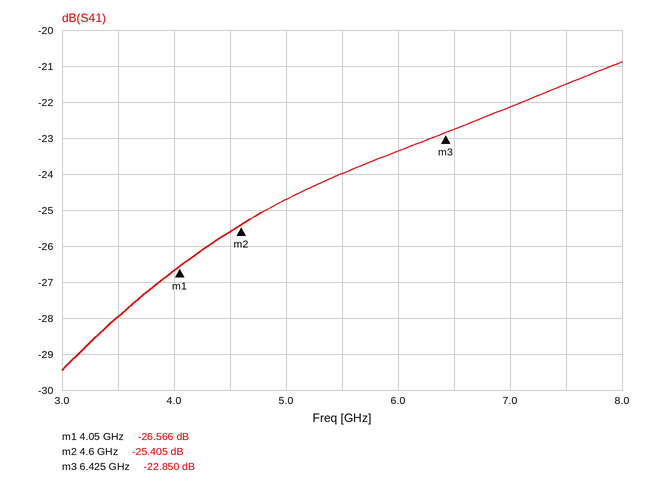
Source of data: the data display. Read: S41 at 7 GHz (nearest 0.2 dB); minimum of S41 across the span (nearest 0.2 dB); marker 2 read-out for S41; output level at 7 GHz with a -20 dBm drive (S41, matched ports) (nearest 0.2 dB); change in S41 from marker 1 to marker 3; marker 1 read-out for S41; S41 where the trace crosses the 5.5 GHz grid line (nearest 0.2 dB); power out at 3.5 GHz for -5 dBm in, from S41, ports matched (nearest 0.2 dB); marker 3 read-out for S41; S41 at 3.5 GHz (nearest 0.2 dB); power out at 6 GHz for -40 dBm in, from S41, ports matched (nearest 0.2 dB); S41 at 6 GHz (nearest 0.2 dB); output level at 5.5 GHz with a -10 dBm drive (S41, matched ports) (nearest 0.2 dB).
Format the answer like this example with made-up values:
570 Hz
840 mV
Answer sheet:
-22.2 dB
-29.4 dB
-25.405 dB
-42.2 dBm
3.716 dB
-26.566 dB
-24.0 dB
-33.0 dBm
-22.850 dB
-28.0 dB
-63.4 dBm
-23.4 dB
-34.0 dBm
